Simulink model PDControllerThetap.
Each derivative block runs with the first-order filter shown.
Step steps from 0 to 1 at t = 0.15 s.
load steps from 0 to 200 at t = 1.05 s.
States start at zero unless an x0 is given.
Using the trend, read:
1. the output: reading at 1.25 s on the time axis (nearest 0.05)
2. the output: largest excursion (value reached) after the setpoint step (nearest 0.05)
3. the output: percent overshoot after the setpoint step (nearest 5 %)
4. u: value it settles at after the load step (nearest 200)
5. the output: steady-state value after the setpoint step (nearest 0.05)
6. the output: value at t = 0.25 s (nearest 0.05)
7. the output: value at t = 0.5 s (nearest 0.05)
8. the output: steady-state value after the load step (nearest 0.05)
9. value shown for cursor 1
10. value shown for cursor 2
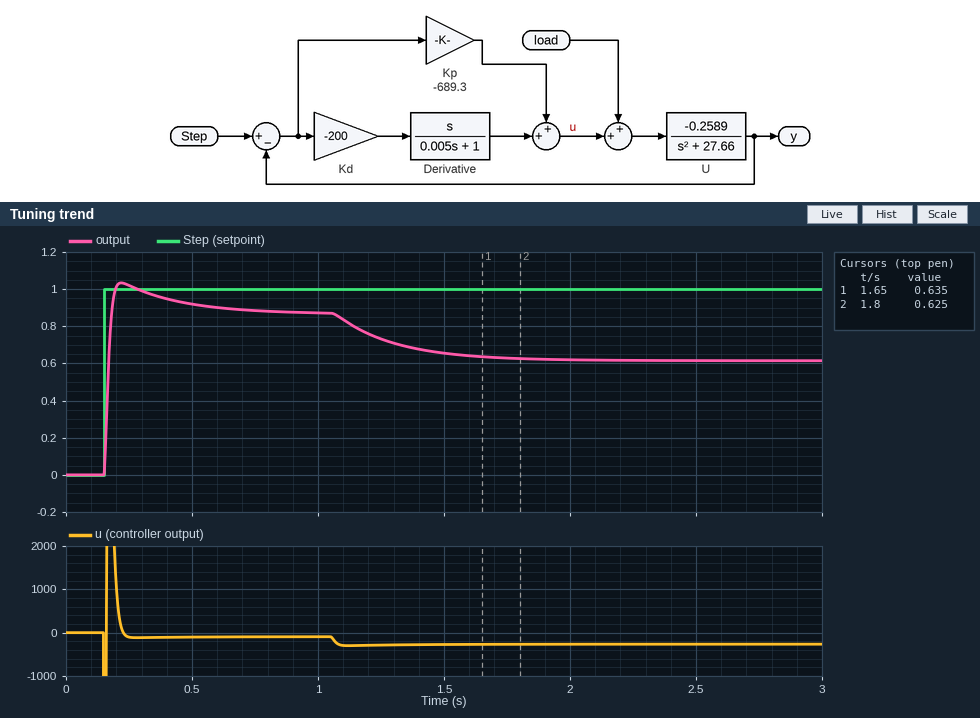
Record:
0.75
1.05
20 %
-200
0.85
1.00
0.90
0.60
0.635
0.625
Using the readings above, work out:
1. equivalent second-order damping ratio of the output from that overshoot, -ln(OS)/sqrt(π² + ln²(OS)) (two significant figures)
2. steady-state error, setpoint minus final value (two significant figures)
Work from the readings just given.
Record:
0.46
0.15
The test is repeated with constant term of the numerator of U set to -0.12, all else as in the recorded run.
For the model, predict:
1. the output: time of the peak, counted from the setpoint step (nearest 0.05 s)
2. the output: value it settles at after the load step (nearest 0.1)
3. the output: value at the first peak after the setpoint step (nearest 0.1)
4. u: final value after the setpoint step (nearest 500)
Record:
0.15 s
0.5
1.0
0
